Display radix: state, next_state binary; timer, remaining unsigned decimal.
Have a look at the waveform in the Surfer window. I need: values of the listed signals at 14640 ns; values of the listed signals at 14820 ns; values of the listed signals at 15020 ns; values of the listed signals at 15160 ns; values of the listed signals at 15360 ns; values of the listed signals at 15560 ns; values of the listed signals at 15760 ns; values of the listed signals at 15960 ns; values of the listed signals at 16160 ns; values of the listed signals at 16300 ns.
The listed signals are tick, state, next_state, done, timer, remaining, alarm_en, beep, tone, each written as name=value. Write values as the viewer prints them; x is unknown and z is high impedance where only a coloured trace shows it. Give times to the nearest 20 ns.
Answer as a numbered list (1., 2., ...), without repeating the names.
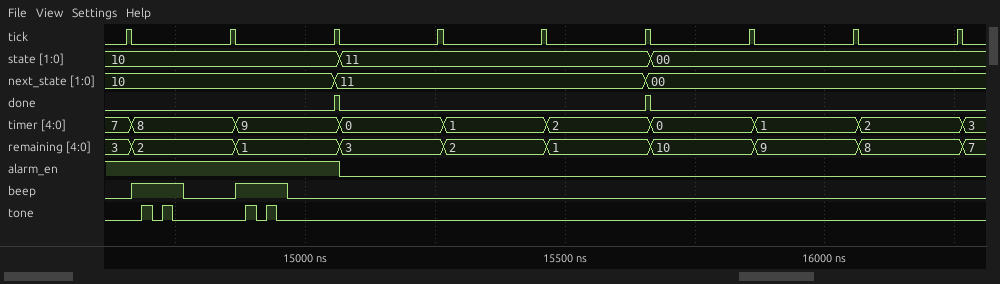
1. tick=0, state=10, next_state=10, done=0, timer=7, remaining=3, alarm_en=1, beep=0, tone=0
2. tick=0, state=10, next_state=10, done=0, timer=8, remaining=2, alarm_en=1, beep=0, tone=0
3. tick=0, state=10, next_state=10, done=0, timer=9, remaining=1, alarm_en=1, beep=0, tone=0
4. tick=0, state=11, next_state=11, done=0, timer=0, remaining=3, alarm_en=0, beep=0, tone=0
5. tick=0, state=11, next_state=11, done=0, timer=1, remaining=2, alarm_en=0, beep=0, tone=0
6. tick=0, state=11, next_state=11, done=0, timer=2, remaining=1, alarm_en=0, beep=0, tone=0
7. tick=0, state=00, next_state=00, done=0, timer=0, remaining=10, alarm_en=0, beep=0, tone=0
8. tick=0, state=00, next_state=00, done=0, timer=1, remaining=9, alarm_en=0, beep=0, tone=0
9. tick=0, state=00, next_state=00, done=0, timer=2, remaining=8, alarm_en=0, beep=0, tone=0
10. tick=0, state=00, next_state=00, done=0, timer=3, remaining=7, alarm_en=0, beep=0, tone=0
